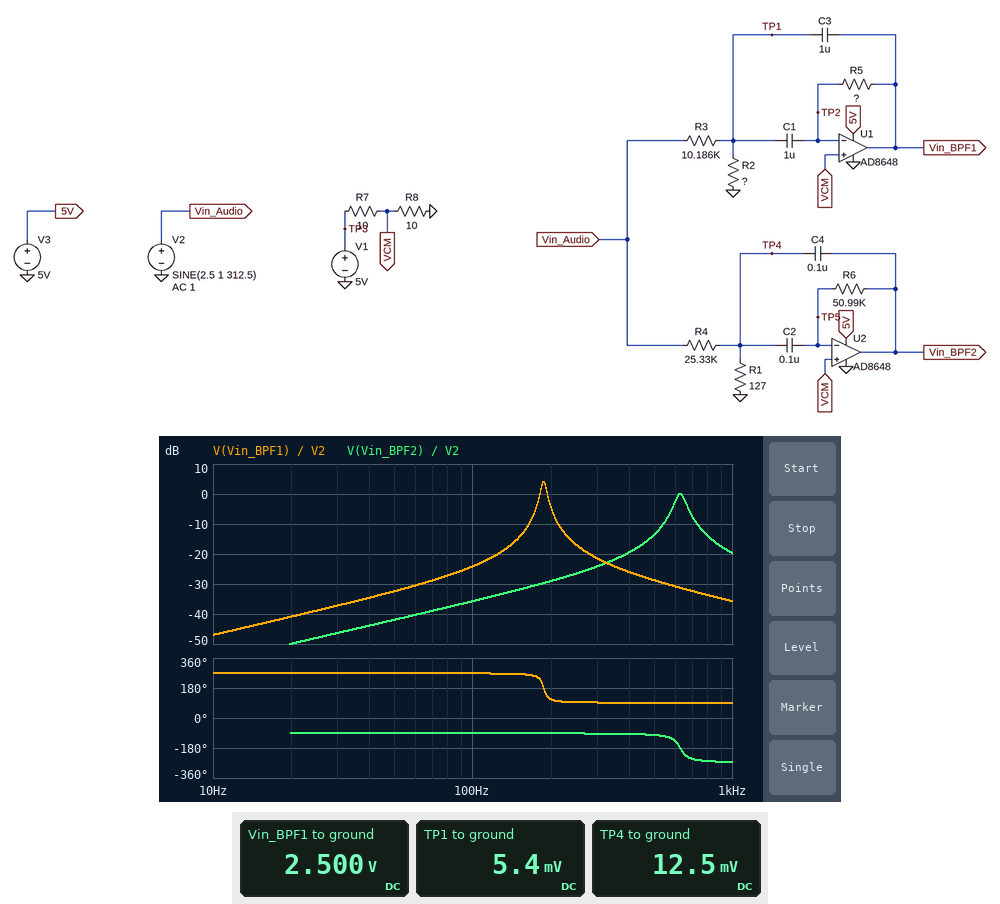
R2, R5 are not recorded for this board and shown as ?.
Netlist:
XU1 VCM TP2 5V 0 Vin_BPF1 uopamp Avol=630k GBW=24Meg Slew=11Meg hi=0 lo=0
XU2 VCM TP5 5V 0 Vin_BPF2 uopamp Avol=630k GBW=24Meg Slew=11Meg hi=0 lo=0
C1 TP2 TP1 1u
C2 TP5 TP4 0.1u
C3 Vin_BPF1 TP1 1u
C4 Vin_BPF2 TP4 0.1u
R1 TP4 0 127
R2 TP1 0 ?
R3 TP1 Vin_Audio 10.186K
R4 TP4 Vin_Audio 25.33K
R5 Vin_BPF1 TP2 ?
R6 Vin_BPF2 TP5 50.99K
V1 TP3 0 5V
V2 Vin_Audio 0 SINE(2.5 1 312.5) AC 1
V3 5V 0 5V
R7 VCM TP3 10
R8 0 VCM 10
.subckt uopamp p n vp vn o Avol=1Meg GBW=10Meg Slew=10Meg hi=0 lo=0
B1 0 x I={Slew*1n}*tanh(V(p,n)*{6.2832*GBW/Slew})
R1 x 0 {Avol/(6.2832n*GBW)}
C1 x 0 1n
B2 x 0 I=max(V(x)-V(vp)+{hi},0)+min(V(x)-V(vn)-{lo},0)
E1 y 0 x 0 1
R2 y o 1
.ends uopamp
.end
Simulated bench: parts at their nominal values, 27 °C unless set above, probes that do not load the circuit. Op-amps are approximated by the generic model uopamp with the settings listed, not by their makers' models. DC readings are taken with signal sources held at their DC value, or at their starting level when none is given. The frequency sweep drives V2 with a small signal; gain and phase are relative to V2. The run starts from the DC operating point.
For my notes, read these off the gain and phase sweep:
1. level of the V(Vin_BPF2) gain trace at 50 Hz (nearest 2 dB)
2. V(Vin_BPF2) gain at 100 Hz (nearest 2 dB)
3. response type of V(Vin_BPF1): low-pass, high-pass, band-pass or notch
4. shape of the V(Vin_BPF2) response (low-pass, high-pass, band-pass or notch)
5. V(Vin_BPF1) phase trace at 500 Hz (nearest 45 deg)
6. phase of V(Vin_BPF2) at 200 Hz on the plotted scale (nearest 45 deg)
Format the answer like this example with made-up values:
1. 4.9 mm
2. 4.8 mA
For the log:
1. -42 dB
2. -36 dB
3. band-pass
4. band-pass
5. 90 deg
6. -90 deg
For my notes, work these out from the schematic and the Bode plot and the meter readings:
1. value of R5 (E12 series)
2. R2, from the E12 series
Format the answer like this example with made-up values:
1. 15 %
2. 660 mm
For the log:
1. 33 kΩ
2. 22 Ω
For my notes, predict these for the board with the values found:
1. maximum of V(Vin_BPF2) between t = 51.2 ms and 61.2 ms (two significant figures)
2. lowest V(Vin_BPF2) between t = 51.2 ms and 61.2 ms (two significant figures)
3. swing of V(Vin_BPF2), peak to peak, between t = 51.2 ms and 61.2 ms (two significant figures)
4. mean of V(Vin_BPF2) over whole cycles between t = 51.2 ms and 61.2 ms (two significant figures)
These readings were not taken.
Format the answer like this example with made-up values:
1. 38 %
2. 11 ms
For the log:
1. 2.6 V
2. 2.4 V
3. 130 mV
4. 2.5 V
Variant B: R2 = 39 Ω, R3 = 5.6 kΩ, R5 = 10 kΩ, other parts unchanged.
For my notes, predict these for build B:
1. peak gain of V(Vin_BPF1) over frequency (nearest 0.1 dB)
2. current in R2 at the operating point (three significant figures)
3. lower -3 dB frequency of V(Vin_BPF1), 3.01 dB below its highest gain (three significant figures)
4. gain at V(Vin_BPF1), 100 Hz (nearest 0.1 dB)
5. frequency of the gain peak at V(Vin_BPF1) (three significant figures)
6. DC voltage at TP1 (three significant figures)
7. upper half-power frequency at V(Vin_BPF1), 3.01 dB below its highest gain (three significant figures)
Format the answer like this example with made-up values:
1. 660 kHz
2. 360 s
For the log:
1. -1.0 dB
2. 443 µA
3. 240 Hz
4. -25.8 dB
5. 256 Hz
6. 17.3 mV
7. 272 Hz
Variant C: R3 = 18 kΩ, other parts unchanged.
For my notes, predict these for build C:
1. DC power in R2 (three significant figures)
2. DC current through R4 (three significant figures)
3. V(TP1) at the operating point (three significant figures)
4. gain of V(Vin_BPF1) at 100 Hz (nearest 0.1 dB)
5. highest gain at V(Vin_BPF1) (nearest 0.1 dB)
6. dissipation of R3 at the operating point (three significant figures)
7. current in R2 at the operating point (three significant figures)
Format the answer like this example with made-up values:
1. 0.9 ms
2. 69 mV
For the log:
1. 423 nW
2. 98.2 µA
3. 3.05 mV
4. -29.0 dB
5. -0.8 dB
6. 346 µW
7. 139 µA
